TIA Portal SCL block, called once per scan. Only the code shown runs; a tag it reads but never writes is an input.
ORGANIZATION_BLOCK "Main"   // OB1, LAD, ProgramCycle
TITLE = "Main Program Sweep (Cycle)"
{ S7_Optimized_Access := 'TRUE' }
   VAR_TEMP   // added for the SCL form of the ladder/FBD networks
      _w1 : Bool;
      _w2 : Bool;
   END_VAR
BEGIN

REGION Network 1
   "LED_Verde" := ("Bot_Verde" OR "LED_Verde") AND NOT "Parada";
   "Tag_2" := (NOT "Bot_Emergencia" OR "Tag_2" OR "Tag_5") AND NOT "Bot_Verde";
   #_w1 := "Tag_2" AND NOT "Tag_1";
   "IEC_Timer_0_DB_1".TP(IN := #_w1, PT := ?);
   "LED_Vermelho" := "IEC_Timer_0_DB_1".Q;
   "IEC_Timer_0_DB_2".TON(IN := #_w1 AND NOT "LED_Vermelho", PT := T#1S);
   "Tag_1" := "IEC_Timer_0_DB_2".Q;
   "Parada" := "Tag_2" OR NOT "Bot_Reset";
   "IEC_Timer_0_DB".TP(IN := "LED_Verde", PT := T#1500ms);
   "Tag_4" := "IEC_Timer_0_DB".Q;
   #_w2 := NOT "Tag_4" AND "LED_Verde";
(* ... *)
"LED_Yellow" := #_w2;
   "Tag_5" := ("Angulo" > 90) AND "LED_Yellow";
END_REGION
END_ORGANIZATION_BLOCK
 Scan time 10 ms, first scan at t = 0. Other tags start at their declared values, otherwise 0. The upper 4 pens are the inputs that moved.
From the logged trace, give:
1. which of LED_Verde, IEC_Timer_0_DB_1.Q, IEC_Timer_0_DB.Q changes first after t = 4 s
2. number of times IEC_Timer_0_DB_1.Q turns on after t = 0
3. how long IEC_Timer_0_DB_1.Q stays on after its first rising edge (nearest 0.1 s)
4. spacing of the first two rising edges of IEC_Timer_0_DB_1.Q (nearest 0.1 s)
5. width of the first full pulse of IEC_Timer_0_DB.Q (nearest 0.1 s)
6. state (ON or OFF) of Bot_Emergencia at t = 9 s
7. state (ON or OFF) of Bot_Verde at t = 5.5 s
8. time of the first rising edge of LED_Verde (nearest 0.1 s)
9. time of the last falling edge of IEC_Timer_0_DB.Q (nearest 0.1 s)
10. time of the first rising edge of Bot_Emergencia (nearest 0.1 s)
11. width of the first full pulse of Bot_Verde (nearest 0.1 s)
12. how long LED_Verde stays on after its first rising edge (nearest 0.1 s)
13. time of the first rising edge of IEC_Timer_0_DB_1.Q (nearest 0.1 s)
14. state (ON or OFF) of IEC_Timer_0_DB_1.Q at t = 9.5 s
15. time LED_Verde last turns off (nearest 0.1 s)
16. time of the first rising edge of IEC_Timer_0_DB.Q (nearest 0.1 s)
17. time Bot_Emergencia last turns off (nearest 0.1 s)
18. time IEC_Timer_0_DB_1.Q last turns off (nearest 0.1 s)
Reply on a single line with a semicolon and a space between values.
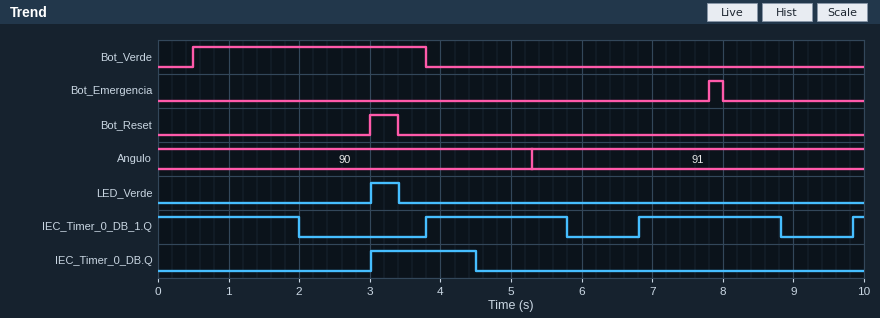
IEC_Timer_0_DB.Q; 3; 2.0 s; 3.0 s; 1.5 s; OFF; OFF; 3.0 s; 4.5 s; 7.8 s; 3.3 s; 0.4 s; 3.8 s; OFF; 3.4 s; 3.0 s; 8.0 s; 8.8 s
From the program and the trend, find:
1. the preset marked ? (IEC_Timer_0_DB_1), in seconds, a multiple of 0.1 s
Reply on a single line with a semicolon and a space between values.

2.0 s
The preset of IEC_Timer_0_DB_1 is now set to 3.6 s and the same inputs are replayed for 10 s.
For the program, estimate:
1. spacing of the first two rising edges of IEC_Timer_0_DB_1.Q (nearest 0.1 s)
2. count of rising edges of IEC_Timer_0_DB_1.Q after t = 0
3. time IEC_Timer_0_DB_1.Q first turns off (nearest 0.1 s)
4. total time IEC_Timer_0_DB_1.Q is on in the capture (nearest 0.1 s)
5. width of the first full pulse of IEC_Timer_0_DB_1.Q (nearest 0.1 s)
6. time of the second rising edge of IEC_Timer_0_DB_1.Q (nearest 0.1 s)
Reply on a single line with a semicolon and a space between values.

4.6 s; 2; 3.6 s; 8.8 s; 3.6 s; 8.4 s
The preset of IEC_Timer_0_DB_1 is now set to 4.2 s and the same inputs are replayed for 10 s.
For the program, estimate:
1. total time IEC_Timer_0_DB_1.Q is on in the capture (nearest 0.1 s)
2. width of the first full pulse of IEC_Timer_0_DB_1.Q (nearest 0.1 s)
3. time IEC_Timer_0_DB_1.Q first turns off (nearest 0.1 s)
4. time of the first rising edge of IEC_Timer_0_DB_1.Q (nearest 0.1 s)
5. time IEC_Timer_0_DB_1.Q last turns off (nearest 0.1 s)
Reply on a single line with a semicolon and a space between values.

8.4 s; 4.2 s; 4.2 s; 5.2 s; 9.4 s
